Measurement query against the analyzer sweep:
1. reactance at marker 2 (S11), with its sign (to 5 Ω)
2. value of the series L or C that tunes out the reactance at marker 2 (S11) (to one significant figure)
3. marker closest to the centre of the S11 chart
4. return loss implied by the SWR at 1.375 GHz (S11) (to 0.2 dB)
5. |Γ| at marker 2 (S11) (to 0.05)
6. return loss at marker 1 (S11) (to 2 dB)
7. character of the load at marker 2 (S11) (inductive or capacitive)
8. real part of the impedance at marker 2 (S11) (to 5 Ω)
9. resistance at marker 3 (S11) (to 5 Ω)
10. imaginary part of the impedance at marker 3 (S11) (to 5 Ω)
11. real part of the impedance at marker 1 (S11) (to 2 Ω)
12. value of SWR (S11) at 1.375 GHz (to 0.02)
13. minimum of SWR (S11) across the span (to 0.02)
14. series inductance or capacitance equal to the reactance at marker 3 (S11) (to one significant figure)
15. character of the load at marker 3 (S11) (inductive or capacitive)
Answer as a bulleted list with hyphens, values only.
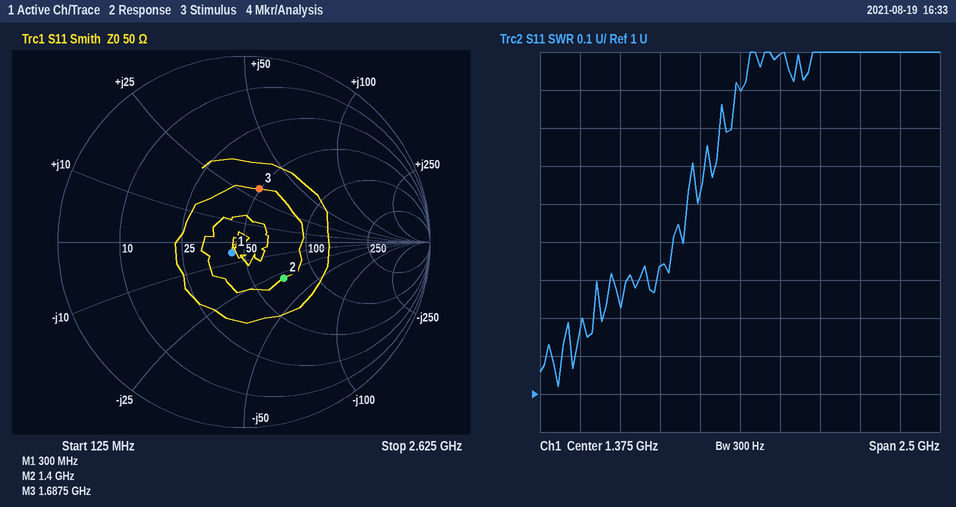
- -30 Ω
- 3 nH
- marker 1
- 10.8 dB
- 0.30
- 22 dB
- capacitive
- 70 Ω
- 50 Ω
- +30 Ω
- 44 Ω
- 1.80
- 1.02
- 3 nH
- inductive
